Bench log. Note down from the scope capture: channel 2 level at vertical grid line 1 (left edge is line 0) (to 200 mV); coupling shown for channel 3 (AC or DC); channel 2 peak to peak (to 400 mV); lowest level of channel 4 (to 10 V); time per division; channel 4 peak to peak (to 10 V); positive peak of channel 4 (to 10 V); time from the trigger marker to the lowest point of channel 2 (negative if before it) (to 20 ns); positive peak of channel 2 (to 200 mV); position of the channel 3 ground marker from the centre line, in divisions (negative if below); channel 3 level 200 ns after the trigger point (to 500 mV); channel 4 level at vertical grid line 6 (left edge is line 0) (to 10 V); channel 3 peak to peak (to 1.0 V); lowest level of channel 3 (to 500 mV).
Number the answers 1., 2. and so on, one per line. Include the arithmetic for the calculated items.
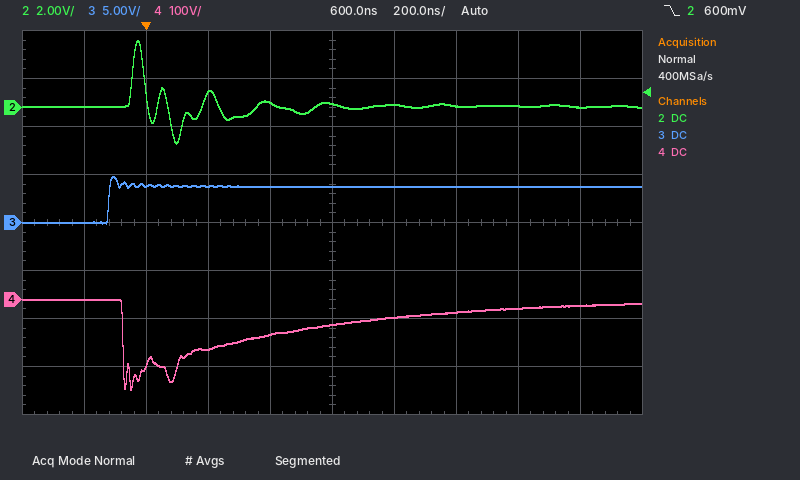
1. 0.0 V
2. DC
3. 4.4 V
4. -190 V
5. 200 ns
6. 0 V − (-190 V) = 190 V
7. 0 V
8. +100 ns
9. 2.8 V
10. 0.0 div
11. 4.0 V
12. -40 V
13. 5.0 V
14. 0.0 V
